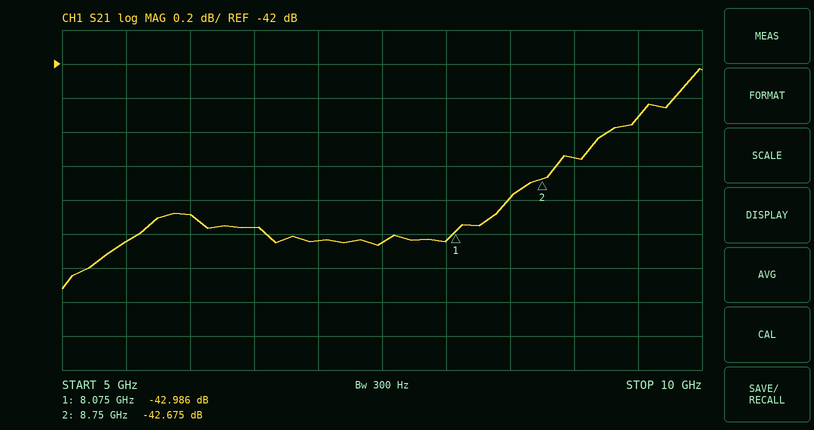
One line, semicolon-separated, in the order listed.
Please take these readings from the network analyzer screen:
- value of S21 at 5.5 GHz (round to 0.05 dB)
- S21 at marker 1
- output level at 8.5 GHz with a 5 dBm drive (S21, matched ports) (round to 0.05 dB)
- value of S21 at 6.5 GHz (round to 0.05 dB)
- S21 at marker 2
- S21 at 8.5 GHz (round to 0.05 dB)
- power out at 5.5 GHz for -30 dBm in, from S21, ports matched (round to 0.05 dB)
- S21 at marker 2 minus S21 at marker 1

-43.05 dB; -42.986 dB; -37.80 dBm; -42.95 dB; -42.675 dB; -42.80 dB; -73.05 dBm; 0.311 dB
